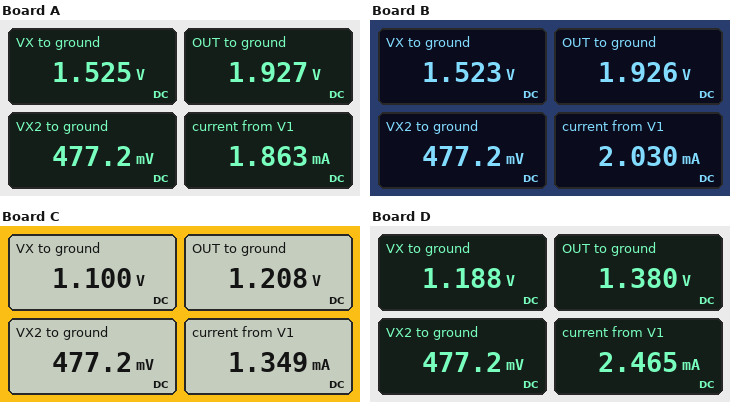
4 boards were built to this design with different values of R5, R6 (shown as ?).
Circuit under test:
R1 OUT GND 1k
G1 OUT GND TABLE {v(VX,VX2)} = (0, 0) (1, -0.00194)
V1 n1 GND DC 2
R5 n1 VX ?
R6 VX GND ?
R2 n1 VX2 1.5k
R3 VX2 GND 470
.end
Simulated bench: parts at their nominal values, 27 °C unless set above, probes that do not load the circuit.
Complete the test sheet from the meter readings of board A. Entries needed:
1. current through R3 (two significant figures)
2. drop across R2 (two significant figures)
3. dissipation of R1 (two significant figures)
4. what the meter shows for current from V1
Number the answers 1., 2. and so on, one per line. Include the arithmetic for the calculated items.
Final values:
1. (477.2 mV) / 470 Ω = 1.0 mA
2. 2 V - 477.2 mV = 1.5 V
3. (1.927 V)^2 / 1 kΩ = 3.7 mW
4. 1.863 mA
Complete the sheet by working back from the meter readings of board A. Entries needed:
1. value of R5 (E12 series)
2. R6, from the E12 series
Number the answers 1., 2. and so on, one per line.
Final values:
1. 560 Ω
2. 1.8 kΩ
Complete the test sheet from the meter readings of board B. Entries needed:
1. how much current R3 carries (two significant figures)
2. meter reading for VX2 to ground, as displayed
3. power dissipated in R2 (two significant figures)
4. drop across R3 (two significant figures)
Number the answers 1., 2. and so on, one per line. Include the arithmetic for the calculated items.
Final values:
1. (477.2 mV) / 470 Ω = 1.0 mA
2. 477.2 mV
3. (2 V - 477.2 mV)^2 / 1.5 kΩ = 1.5 mW
4. 477.2 mV = 480 mV
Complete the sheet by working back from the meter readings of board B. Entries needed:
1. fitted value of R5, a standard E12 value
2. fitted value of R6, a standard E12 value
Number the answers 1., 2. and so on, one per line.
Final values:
1. 470 Ω
2. 1.5 kΩ
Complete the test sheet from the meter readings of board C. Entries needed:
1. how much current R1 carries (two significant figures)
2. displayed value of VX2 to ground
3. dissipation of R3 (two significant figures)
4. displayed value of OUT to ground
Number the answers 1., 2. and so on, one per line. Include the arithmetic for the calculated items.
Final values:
1. (1.208 V) / 1 kΩ = 1.2 mA
2. 477.2 mV
3. (477.2 mV)^2 / 470 Ω = 480 µW
4. 1.208 V
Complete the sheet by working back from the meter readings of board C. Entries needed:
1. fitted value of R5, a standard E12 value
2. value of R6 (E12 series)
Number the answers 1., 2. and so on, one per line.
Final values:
1. 2.7 kΩ
2. 3.3 kΩ
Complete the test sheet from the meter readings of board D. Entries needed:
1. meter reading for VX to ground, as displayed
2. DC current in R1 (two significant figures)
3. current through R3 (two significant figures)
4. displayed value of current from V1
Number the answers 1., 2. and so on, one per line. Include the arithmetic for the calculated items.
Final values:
1. 1.188 V
2. (1.38 V) / 1 kΩ = 1.4 mA
3. (477.2 mV) / 470 Ω = 1.0 mA
4. 2.465 mA
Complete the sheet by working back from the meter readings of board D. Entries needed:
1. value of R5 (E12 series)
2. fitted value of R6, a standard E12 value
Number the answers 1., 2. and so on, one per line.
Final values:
1. 560 Ω
2. 820 Ω
